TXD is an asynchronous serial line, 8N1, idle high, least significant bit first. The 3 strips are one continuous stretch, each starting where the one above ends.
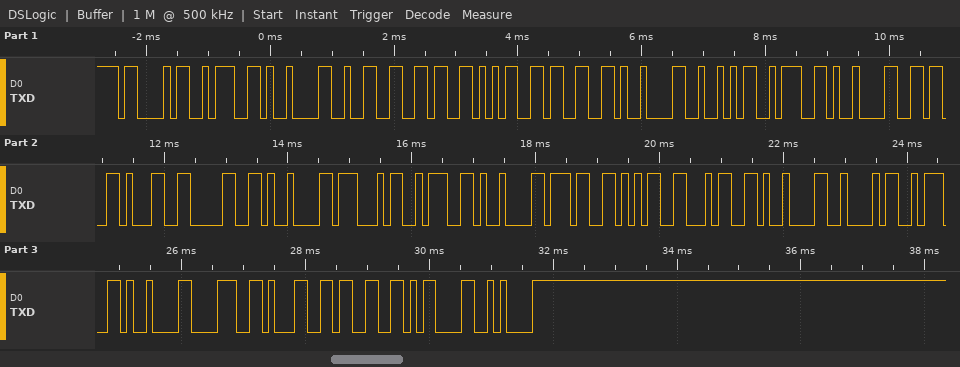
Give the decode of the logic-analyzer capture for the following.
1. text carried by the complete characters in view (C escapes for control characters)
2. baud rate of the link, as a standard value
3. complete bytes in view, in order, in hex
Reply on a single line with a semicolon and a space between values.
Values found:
"C:\t2653\tR:\t610\tG:\t754\tB:\t813\r\n"; 9600 baud; 43 3A 09 32 36 35 33 09 52 3A 09 36 31 30 09 47 3A 09 37 35 34 09 42 3A 09 38 31 33 0D 0A
